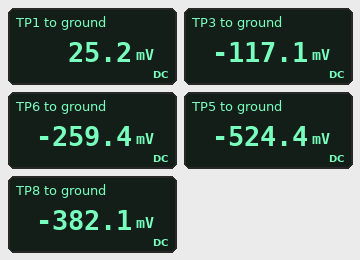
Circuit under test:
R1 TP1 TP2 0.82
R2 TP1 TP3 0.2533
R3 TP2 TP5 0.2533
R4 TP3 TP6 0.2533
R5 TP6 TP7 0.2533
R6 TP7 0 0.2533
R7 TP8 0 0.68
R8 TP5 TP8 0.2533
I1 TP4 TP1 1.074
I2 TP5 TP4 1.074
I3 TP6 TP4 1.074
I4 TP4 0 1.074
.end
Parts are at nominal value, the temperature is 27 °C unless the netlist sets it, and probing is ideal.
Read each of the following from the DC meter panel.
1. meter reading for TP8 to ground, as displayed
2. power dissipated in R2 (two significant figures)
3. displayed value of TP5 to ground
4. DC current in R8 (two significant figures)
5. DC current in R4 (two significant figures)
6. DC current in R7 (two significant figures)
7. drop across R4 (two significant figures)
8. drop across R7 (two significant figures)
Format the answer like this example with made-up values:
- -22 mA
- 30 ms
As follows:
- -382.1 mV
- 80 mW
- -524.4 mV
- 560 mA
- 560 mA
- 560 mA
- 140 mV
- 380 mV
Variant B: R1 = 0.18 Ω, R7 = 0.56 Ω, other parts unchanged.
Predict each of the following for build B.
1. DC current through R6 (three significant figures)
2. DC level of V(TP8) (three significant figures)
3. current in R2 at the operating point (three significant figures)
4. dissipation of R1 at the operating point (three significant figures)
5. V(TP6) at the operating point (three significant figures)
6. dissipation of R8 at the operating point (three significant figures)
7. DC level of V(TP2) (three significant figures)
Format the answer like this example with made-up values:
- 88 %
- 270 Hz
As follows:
- 627 mA
- -250 mV
- 447 mA
- 70.8 mW
- -318 mV
- 50.5 mW
- -204 mV
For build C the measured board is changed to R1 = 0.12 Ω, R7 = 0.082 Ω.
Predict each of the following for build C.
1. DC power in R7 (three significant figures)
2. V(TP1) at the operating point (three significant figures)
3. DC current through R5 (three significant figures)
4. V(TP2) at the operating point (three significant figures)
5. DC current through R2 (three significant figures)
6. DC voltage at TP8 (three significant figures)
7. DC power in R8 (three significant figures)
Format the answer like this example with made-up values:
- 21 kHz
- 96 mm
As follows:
- 24.7 mW
- 12.0 mV
- 525 mA
- -51.0 mV
- 549 mA
- -45.0 mV
- 76.3 mW
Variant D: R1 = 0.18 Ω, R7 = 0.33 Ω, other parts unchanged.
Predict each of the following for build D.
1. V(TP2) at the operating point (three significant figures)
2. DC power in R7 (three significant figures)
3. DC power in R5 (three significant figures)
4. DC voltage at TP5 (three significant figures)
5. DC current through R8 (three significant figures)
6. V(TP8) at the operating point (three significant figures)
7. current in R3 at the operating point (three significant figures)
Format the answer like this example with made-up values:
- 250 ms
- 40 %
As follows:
- -144 mV
- 81.6 mW
- 84.2 mW
- -290 mV
- 497 mA
- -164 mV
- 577 mA
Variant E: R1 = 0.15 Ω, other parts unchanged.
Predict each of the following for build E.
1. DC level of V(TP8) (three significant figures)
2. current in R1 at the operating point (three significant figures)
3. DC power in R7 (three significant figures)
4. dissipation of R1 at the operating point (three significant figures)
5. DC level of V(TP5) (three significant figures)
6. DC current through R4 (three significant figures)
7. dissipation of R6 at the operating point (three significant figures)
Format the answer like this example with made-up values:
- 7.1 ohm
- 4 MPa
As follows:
- -283 mV
- 658 mA
- 118 mW
- 65.0 mW
- -388 mV
- 416 mA
- 110 mW
